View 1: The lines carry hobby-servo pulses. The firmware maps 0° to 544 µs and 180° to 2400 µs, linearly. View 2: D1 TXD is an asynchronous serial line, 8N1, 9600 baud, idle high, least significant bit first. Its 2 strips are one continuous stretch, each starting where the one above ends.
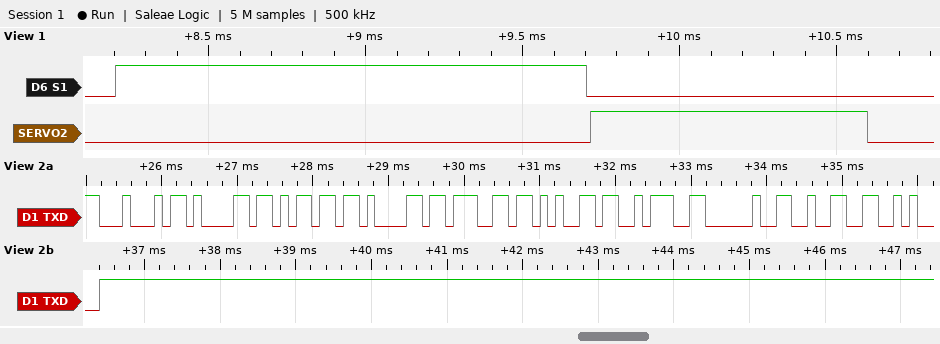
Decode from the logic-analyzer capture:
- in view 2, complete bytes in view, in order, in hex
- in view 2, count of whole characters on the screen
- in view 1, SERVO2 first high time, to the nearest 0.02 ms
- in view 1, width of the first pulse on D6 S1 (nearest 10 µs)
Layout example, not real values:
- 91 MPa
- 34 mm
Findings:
- 44 61 6D 61 67 65 3A 20 32 0A
- 10
- 0.88 ms
- 1500 µs
